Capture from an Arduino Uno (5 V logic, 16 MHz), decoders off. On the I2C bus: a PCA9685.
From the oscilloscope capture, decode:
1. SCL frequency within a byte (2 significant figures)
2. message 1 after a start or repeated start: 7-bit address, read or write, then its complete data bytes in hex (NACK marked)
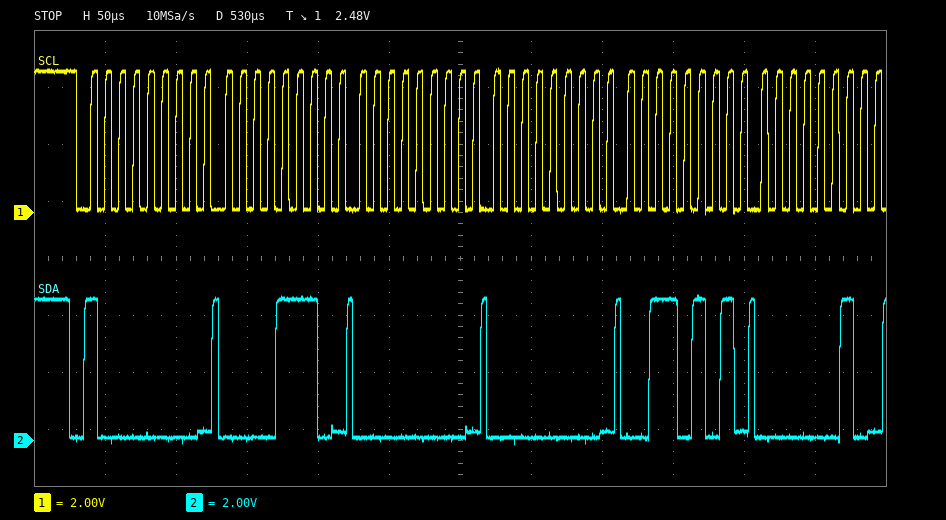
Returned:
100 kHz
0x40 write: 0E 00 00 35 02
